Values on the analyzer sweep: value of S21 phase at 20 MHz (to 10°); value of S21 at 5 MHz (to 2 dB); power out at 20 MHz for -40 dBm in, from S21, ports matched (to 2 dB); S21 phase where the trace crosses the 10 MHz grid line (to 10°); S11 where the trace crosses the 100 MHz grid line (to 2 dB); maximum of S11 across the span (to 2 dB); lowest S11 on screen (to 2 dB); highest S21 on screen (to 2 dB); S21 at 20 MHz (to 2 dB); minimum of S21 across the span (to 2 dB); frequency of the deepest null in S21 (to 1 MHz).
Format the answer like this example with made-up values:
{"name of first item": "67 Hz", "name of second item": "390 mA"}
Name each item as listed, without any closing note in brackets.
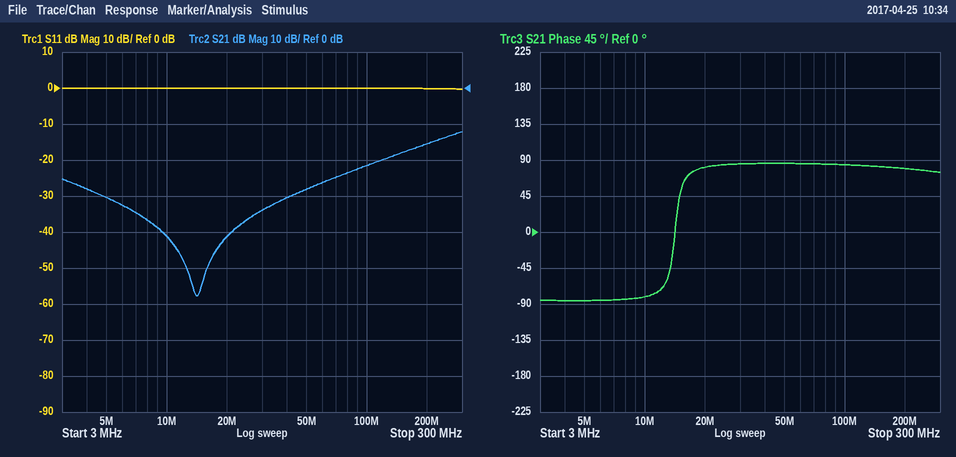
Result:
{"value of S21 phase at 20 MHz": "80°", "value of S21 at 5 MHz": "-30 dB", "power out at 20 MHz for -40 dBm in, from S21, ports matched": "-82 dBm", "S21 phase where the trace crosses the 10 MHz grid line": "-80°", "S11 where the trace crosses the 100 MHz grid line": "0 dB", "maximum of S11 across the span": "0 dB", "lowest S11 on screen": "0 dB", "highest S21 on screen": "-12 dB", "S21 at 20 MHz": "-42 dB", "minimum of S21 across the span": "-58 dB", "frequency of the deepest null in S21": "14 MHz"}
